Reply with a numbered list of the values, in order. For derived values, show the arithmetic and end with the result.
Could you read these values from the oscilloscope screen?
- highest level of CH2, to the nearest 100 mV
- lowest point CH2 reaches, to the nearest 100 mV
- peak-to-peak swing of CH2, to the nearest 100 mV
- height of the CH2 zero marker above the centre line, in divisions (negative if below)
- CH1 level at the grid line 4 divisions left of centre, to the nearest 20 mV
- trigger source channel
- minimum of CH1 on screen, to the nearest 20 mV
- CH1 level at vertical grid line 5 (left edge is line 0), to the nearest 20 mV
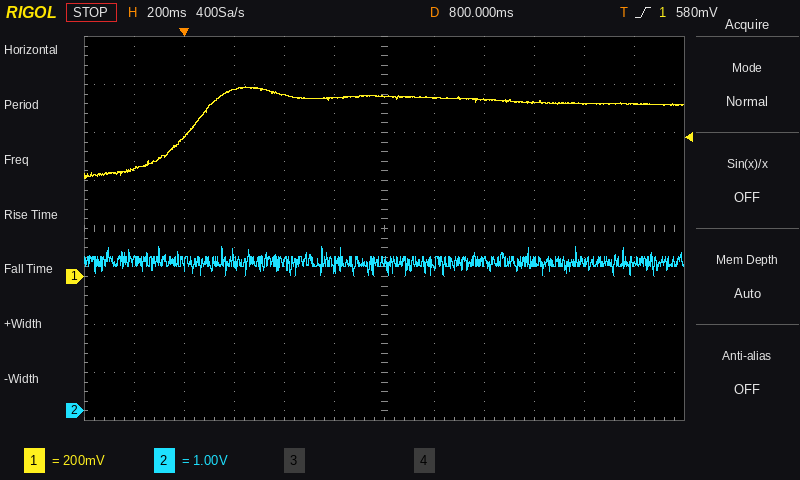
1. 3.4 V
2. 2.8 V
3. 3.4 V − (2.8 V) = 600 mV
4. -3.8 div
5. 580 mV
6. CH1
7. 400 mV
8. 740 mV
